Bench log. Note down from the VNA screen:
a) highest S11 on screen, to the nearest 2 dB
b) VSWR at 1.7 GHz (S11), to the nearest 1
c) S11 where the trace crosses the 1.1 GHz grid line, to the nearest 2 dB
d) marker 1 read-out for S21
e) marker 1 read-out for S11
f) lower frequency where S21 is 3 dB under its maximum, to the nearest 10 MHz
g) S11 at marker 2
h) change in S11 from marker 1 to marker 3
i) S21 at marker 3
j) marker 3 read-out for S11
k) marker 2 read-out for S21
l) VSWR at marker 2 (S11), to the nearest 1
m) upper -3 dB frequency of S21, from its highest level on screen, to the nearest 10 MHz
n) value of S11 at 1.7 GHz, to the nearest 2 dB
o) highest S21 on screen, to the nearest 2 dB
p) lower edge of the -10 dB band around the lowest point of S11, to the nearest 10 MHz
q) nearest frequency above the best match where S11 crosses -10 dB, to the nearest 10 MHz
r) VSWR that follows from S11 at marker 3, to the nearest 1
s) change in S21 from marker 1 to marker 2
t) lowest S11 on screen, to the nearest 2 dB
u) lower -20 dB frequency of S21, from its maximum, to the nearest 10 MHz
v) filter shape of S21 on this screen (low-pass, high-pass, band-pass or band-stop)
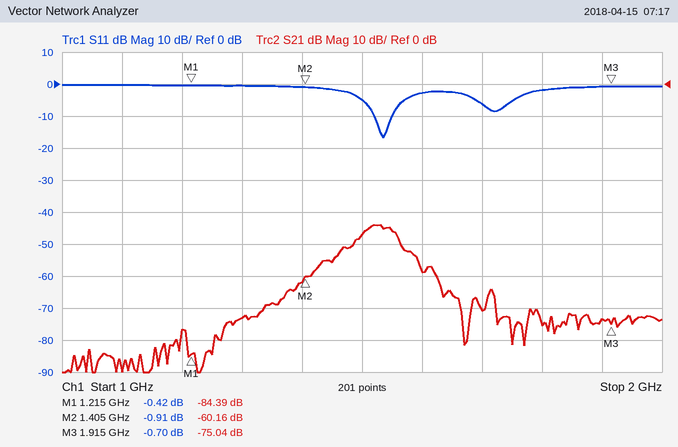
0 dB
3
0 dB
-84.39 dB
-0.42 dB
1.50 GHz
-0.91 dB
-0.28 dB
-75.04 dB
-0.70 dB
-60.16 dB
19
1.56 GHz
-6 dB
-44 dB
1.52 GHz
1.55 GHz
25
24.23 dB
-16 dB
1.39 GHz
band-pass
